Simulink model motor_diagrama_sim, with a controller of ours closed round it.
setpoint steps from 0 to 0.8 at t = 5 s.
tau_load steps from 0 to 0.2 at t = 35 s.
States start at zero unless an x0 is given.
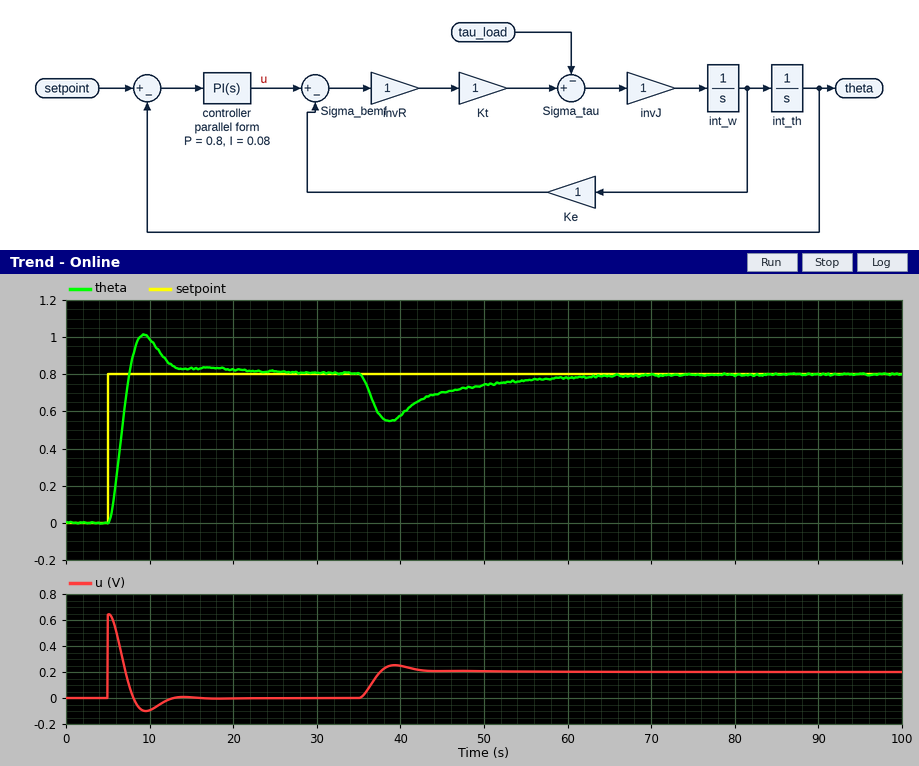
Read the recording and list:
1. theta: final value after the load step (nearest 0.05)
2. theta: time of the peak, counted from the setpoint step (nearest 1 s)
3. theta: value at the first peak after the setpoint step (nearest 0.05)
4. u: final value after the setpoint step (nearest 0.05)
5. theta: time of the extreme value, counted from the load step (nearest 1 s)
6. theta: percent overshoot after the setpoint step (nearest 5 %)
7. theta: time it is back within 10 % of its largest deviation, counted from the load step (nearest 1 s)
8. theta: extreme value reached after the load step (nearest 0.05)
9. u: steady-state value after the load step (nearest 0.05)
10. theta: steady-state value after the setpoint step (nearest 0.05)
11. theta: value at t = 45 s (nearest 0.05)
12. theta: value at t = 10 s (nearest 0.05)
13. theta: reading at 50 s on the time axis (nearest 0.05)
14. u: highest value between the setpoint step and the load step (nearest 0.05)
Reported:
0.80
4 s
1.00
0.00
4 s
25 %
22 s
0.55
0.20
0.80
0.70
1.00
0.75
0.65
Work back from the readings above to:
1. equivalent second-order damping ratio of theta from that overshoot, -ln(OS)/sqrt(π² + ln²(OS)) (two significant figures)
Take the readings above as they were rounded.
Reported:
0.40
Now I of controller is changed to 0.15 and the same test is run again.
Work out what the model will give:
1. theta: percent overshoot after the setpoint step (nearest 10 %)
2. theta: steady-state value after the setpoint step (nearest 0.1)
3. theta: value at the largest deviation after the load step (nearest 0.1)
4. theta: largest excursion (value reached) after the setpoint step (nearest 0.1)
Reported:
40 %
0.8
0.6
1.1
